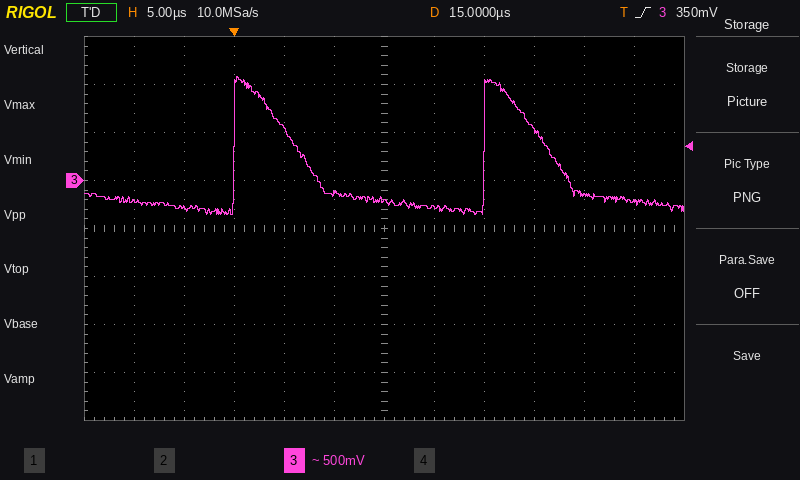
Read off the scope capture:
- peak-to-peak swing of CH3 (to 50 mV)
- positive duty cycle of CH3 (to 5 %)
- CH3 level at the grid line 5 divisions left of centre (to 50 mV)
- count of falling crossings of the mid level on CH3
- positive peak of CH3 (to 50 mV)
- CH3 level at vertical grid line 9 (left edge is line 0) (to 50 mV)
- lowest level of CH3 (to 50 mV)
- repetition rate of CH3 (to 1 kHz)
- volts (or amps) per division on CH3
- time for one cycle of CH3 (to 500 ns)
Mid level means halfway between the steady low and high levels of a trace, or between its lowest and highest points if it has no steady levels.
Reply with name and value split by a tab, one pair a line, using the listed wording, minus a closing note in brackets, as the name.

peak-to-peak swing of CH3	1.45 V
positive duty cycle of CH3	25 %
CH3 level at the grid line 5 divisions left of centre	-200 mV
count of falling crossings of the mid level on CH3	2
positive peak of CH3	1.10 V
CH3 level at vertical grid line 9 (left edge is line 0)	550 mV
lowest level of CH3	-350 mV
repetition rate of CH3	40 kHz
volts (or amps) per division on CH3	500 mV
time for one cycle of CH3	25.0 µs
